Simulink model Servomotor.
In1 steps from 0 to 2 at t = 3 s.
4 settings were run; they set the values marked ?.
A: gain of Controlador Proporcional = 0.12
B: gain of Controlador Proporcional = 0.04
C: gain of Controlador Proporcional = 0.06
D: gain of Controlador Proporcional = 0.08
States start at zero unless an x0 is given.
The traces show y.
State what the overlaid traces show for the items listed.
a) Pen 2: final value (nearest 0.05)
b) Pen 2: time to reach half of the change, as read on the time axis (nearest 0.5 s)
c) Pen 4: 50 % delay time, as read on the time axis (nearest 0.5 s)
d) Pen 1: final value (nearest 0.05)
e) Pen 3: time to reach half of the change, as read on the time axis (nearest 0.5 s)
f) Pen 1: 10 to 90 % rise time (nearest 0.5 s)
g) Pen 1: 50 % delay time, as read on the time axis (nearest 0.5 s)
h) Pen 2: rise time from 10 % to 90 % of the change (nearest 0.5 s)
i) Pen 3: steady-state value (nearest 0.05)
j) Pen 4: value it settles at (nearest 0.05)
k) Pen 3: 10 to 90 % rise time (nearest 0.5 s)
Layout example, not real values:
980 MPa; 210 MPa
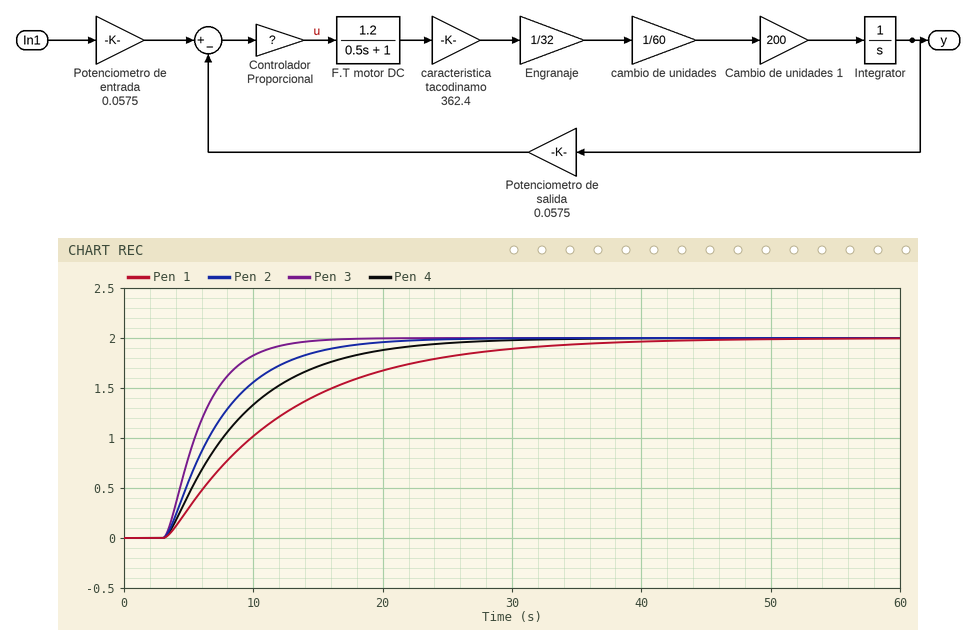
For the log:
2.00; 6.5 s; 7.5 s; 2.00; 5.5 s; 20.0 s; 10.0 s; 9.5 s; 2.00; 2.00; 6.0 s
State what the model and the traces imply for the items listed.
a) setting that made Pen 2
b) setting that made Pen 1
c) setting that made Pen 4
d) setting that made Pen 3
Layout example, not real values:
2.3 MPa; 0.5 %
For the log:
D; B; C; A
